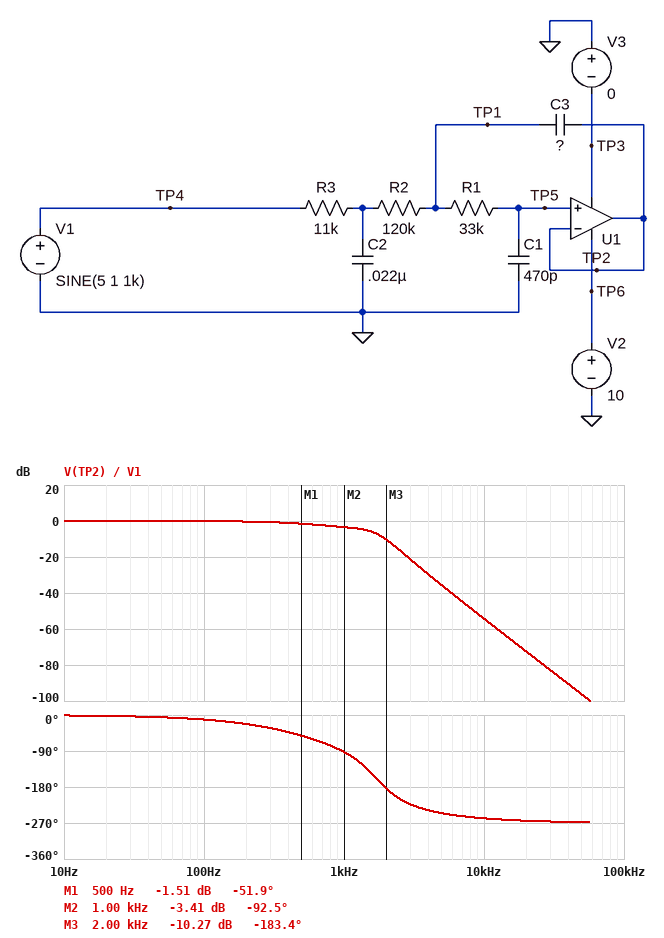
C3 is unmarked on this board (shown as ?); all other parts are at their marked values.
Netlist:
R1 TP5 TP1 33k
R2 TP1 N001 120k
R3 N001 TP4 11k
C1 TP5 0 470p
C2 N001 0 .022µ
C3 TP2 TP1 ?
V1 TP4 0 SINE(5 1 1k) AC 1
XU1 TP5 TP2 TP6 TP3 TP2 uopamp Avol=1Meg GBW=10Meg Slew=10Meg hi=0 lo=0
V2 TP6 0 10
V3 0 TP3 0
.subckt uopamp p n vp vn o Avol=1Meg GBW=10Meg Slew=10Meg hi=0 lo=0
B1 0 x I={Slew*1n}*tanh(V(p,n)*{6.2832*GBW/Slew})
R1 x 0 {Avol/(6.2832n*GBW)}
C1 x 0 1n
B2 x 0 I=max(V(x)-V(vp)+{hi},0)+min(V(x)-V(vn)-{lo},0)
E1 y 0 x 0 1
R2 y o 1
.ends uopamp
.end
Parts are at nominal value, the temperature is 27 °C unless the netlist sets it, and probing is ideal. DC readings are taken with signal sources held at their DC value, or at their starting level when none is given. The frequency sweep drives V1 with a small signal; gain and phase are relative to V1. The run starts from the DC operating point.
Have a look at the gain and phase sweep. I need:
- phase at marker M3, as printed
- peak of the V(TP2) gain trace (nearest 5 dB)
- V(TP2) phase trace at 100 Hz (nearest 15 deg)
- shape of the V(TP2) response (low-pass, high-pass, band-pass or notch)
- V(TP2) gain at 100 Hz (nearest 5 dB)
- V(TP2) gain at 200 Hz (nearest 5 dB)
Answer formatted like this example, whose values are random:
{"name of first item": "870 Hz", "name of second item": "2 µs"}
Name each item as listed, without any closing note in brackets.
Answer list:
{"phase at marker M3, as printed": "-183.4 deg", "peak of the V(TP2) gain trace": "0 dB", "V(TP2) phase trace at 100 Hz": "-15 deg", "shape of the V(TP2) response": "low-pass", "V(TP2) gain at 100 Hz": "0 dB", "V(TP2) gain at 200 Hz": "0 dB"}
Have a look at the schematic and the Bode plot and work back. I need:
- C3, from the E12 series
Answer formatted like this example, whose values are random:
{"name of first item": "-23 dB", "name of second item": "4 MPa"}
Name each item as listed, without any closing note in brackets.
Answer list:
{"C3, from the E12 series": "4.7 nF"}
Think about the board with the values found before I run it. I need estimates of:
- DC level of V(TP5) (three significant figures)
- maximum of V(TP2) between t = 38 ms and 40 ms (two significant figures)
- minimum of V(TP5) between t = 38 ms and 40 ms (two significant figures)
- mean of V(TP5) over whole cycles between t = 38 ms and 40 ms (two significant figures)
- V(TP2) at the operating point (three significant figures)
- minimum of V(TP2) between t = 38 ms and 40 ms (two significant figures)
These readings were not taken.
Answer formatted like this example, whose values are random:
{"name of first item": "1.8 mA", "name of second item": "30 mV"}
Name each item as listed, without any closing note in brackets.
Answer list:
{"DC level of V(TP5)": "5.00 V", "maximum of V(TP2) between t = 38 ms and 40 ms": "5.7 V", "minimum of V(TP5) between t = 38 ms and 40 ms": "4.3 V", "mean of V(TP5) over whole cycles between t = 38 ms and 40 ms": "5.0 V", "V(TP2) at the operating point": "5.00 V", "minimum of V(TP2) between t = 38 ms and 40 ms": "4.3 V"}
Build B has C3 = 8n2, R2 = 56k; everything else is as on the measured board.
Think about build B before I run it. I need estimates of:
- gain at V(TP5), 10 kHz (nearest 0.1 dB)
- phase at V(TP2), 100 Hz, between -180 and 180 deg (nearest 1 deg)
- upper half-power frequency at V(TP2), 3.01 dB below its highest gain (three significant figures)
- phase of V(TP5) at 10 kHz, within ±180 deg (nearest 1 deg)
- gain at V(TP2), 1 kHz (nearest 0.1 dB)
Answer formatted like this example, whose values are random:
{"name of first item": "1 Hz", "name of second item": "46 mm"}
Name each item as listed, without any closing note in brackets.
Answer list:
{"gain at V(TP5), 10 kHz": "-52.4 dB", "phase at V(TP2), 100 Hz, between -180 and 180 deg": "-10 deg", "upper half-power frequency at V(TP2), 3.01 dB below its highest gain": "1.01 kHz", "phase of V(TP5) at 10 kHz, within ±180 deg": "100 deg", "gain at V(TP2), 1 kHz": "-3.0 dB"}
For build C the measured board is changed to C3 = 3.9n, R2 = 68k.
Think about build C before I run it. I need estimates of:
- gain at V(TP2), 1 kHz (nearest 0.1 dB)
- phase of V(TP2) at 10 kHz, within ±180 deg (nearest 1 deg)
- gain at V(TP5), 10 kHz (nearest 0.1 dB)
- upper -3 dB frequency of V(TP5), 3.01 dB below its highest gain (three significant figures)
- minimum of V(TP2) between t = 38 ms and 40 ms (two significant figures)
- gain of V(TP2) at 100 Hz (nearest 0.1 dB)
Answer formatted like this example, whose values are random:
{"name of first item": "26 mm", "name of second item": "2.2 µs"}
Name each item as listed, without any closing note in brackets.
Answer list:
{"gain at V(TP2), 1 kHz": "-4.3 dB", "phase of V(TP2) at 10 kHz, within ±180 deg": "105 deg", "gain at V(TP5), 10 kHz": "-47.5 dB", "upper -3 dB frequency of V(TP5), 3.01 dB below its highest gain": "727 Hz", "minimum of V(TP2) between t = 38 ms and 40 ms": "4.4 V", "gain of V(TP2) at 100 Hz": "-0.1 dB"}
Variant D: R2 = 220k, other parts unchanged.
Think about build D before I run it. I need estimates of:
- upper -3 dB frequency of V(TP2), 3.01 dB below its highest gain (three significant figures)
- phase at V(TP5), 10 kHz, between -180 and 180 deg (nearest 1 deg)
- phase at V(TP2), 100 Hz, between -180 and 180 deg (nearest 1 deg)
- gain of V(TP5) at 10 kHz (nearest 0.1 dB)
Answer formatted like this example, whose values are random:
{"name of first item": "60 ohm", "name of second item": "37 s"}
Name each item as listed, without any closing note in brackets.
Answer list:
{"upper -3 dB frequency of V(TP2), 3.01 dB below its highest gain": "870 Hz", "phase at V(TP5), 10 kHz, between -180 and 180 deg": "101 deg", "phase at V(TP2), 100 Hz, between -180 and 180 deg": "-13 deg", "gain of V(TP5) at 10 kHz": "-59.6 dB"}
